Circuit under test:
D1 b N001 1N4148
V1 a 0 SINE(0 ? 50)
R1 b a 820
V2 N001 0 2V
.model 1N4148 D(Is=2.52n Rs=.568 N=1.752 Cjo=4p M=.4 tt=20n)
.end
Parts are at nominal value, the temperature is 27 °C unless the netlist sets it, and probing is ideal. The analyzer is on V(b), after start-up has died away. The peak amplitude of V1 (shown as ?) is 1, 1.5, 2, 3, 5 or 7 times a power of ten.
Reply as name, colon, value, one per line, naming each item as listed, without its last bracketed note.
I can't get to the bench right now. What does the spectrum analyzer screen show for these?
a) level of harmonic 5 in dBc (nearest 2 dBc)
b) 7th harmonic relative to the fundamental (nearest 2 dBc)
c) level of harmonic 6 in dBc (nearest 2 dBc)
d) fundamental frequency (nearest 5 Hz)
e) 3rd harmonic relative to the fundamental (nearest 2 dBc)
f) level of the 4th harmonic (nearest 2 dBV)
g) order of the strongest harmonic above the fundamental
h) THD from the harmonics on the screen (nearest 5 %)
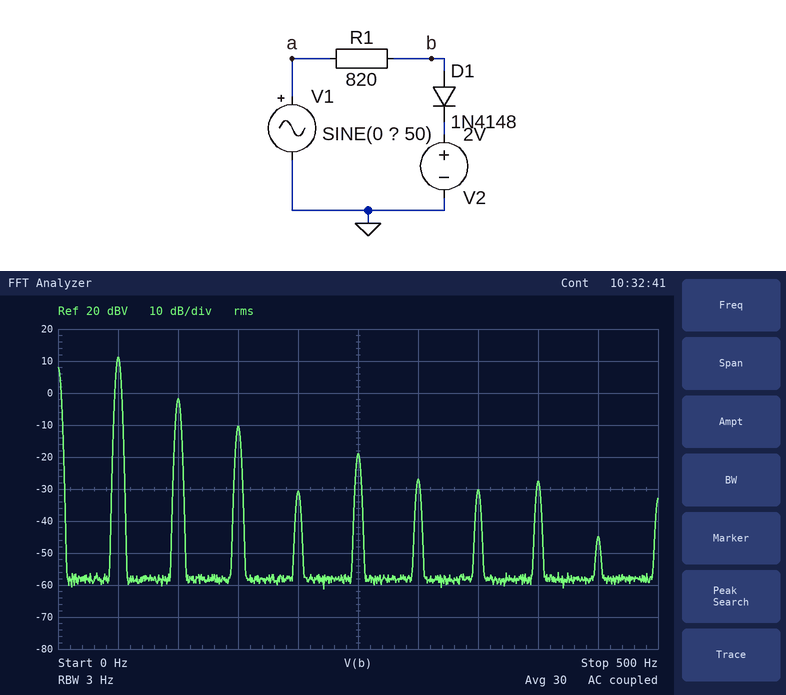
level of harmonic 5 in dBc: -30 dBc
7th harmonic relative to the fundamental: -42 dBc
level of harmonic 6 in dBc: -38 dBc
fundamental frequency: 50 Hz
3rd harmonic relative to the fundamental: -22 dBc
level of the 4th harmonic: -30 dBV
order of the strongest harmonic above the fundamental: 2
THD from the harmonics on the screen: 25 %
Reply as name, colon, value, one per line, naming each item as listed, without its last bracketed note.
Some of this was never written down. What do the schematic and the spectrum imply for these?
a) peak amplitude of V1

peak amplitude of V1: 7 V
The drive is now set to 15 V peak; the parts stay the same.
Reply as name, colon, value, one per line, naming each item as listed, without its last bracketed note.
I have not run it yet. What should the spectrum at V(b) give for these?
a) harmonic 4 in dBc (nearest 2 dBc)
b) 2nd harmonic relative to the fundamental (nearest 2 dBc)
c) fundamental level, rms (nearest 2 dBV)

harmonic 4 in dBc: -26 dBc
2nd harmonic relative to the fundamental: -10 dBc
fundamental level, rms: 16 dBV
